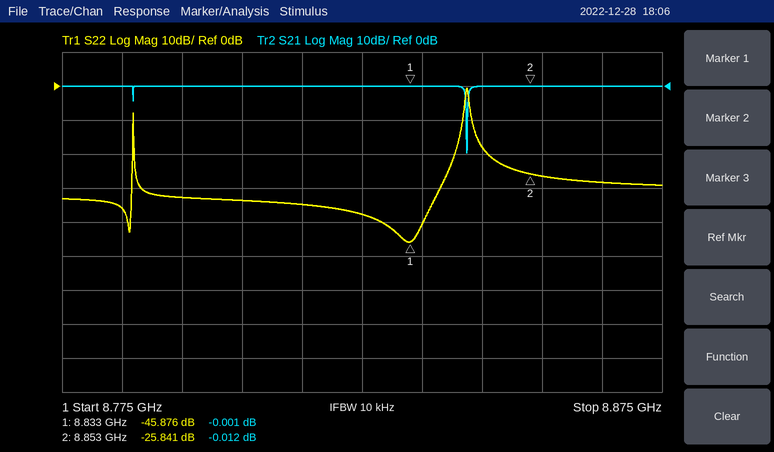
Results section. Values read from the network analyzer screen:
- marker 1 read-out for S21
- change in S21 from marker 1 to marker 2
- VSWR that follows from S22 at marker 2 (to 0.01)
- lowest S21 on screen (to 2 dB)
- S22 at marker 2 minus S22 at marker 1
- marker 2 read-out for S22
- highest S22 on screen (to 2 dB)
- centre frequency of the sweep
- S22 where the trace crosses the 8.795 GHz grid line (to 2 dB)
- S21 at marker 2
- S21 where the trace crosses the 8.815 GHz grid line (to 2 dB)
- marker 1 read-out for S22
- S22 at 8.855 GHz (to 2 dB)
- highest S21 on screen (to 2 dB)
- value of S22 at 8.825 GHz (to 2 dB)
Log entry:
-0.001 dB
-0.011 dB
1.11
-20 dB
20.035 dB
-25.841 dB
0 dB
8.825 GHz
-32 dB
-0.012 dB
0 dB
-45.876 dB
-26 dB
0 dB
-38 dB
